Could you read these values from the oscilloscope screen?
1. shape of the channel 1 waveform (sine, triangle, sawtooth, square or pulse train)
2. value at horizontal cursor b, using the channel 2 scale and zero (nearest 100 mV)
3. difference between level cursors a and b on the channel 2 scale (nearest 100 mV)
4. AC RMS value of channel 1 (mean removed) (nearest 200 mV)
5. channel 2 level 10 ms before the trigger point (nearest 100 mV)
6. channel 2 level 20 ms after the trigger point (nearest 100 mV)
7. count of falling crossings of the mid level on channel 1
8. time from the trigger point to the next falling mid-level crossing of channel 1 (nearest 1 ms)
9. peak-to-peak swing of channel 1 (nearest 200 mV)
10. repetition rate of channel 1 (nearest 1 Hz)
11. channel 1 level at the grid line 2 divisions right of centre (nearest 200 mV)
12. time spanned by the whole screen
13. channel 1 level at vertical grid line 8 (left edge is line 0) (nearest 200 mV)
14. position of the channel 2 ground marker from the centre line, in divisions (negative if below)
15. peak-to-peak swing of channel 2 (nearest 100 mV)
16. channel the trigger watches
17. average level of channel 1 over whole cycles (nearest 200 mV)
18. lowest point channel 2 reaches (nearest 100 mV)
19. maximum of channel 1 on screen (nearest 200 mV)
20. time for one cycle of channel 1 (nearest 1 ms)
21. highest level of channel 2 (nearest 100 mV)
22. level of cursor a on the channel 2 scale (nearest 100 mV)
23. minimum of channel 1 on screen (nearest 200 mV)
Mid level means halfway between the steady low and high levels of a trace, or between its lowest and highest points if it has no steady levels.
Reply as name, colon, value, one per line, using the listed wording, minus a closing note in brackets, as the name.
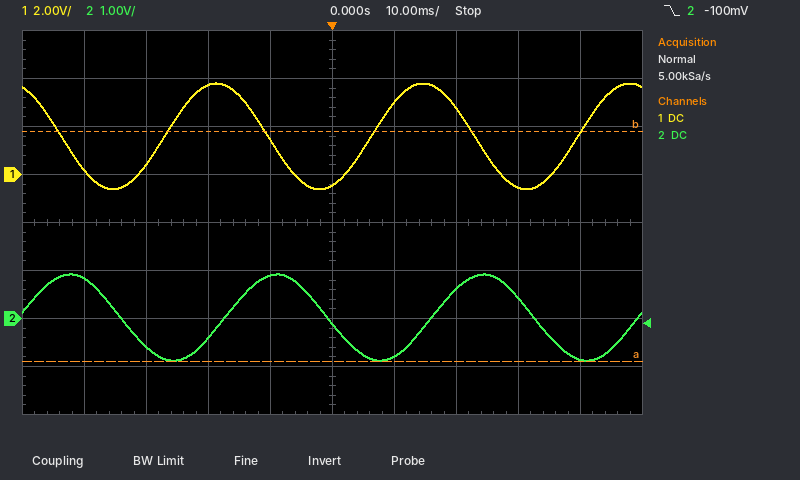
shape of the channel 1 waveform: sine
value at horizontal cursor b, using the channel 2 scale and zero: 3.9 V
difference between level cursors a and b on the channel 2 scale: 4.8 V
AC RMS value of channel 1 (mean removed): 1.6 V
channel 2 level 10 ms before the trigger point: 900 mV
channel 2 level 20 ms after the trigger point: 600 mV
count of falling crossings of the mid level on channel 1: 3
time from the trigger point to the next falling mid-level crossing of channel 1: 23 ms
peak-to-peak swing of channel 1: 4.4 V
repetition rate of channel 1: 30 Hz
channel 1 level at the grid line 2 divisions right of centre: 2.8 V
time spanned by the whole screen: 100 ms
channel 1 level at vertical grid line 8 (left edge is line 0): -600 mV
position of the channel 2 ground marker from the centre line, in divisions: -2.0 div
peak-to-peak swing of channel 2: 1.8 V
channel the trigger watches: channel 2
average level of channel 1 over whole cycles: 1.6 V
lowest point channel 2 reaches: -900 mV
maximum of channel 1 on screen: 3.8 V
time for one cycle of channel 1: 33 ms
highest level of channel 2: 900 mV
level of cursor a on the channel 2 scale: -900 mV
minimum of channel 1 on screen: -600 mV
